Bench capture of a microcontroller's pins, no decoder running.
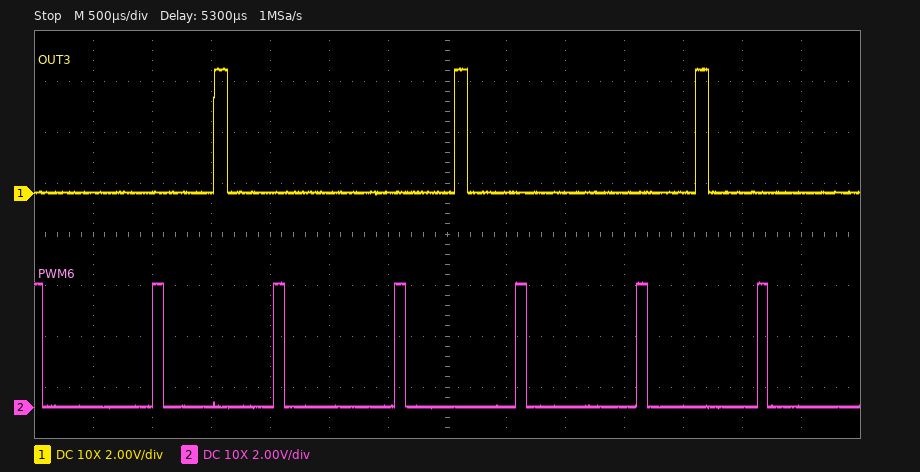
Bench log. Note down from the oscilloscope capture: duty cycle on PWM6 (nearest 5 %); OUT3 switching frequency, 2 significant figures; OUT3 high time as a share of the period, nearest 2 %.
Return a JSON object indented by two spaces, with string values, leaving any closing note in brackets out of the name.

{
  "duty cycle on PWM6": "10 %",
  "OUT3 switching frequency, 2 significant figures": "490 Hz",
  "OUT3 high time as a share of the period, nearest 2 %": "6 %"
}
